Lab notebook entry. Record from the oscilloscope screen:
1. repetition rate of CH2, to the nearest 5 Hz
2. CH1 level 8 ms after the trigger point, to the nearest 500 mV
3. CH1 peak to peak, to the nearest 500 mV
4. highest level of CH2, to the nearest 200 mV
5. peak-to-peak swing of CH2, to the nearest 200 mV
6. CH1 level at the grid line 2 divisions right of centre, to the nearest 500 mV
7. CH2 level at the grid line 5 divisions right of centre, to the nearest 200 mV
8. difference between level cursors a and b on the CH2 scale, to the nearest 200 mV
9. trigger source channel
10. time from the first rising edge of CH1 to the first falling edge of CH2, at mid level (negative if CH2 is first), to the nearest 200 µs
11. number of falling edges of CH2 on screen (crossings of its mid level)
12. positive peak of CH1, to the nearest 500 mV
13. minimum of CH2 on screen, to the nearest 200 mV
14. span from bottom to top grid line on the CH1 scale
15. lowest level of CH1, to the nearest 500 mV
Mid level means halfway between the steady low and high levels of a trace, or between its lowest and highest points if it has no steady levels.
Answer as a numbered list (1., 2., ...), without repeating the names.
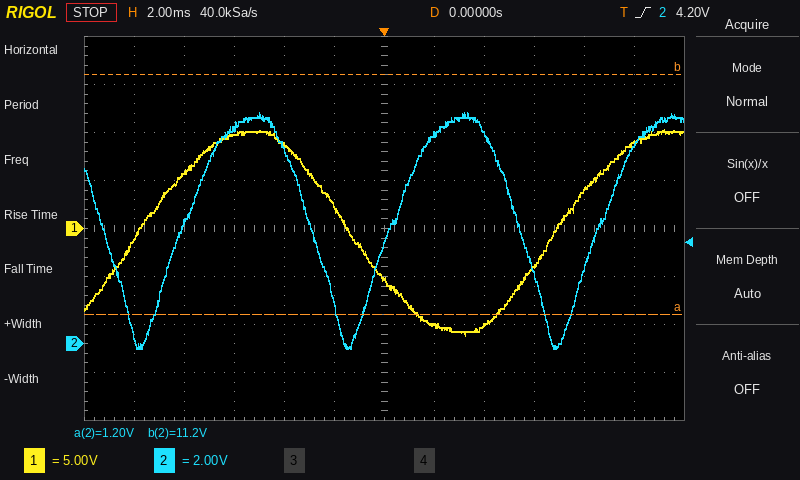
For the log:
1. 120 Hz
2. 4.0 V
3. 21.5 V
4. 9.6 V
5. 9.8 V
6. -10.0 V
7. 8.2 V
8. 10.0 V
9. CH2
10. -1.4 ms
11. 3
12. 10.5 V
13. -200 mV
14. 40 V
15. -11.0 V
